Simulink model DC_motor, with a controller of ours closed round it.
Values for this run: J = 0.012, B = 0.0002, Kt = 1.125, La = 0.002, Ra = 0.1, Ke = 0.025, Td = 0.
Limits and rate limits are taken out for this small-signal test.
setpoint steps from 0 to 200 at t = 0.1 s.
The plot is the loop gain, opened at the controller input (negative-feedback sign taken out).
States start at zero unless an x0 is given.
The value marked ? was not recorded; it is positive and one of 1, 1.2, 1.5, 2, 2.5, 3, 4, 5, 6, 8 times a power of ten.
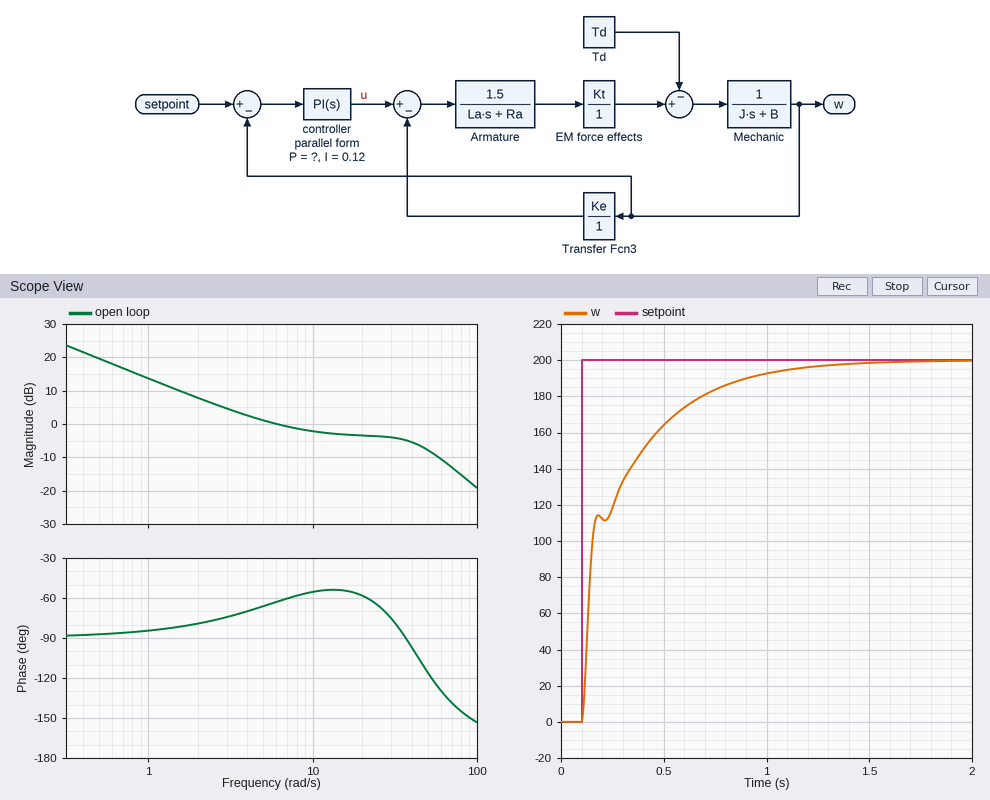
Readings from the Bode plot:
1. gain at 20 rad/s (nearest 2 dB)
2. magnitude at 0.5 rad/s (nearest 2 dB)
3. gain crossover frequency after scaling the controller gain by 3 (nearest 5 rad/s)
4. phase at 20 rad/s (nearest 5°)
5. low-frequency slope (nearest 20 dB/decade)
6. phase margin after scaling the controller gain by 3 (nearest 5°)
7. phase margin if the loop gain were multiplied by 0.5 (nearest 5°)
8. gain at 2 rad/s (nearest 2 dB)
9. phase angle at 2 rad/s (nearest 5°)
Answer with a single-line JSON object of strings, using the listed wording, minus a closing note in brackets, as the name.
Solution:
{"gain at 20 rad/s": "-4 dB", "magnitude at 0.5 rad/s": "20 dB", "gain crossover frequency after scaling the controller gain by 3": "55 rad/s", "phase at 20 rad/s": "-60°", "low-frequency slope": "-20 dB/decade", "phase margin after scaling the controller gain by 3": "55°", "phase margin if the loop gain were multiplied by 0.5": "105°", "gain at 2 rad/s": "8 dB", "phase angle at 2 rad/s": "-80°"}
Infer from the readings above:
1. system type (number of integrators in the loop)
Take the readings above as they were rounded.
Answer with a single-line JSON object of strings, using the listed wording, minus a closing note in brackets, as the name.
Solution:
{"system type": "1"}
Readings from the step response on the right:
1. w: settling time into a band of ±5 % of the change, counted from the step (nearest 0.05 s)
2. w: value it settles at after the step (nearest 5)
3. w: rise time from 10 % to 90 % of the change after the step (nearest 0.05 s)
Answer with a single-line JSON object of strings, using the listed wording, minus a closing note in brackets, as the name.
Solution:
{"w: settling time into a band of ±5 % of the change, counted from the step": "0.80 s", "w: value it settles at after the step": "200", "w: rise time from 10 % to 90 % of the change after the step": "0.55 s"}
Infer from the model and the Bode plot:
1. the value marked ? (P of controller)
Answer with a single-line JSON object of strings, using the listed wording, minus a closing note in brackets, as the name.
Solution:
{"the value marked ?": "0.015"}
